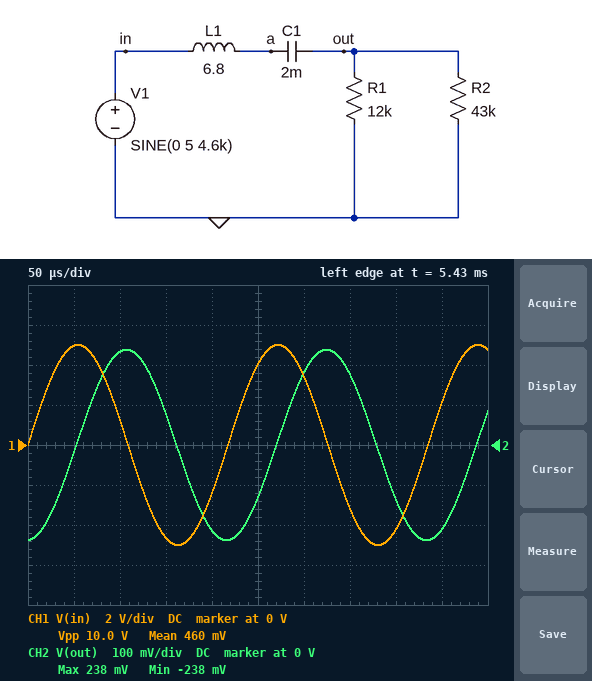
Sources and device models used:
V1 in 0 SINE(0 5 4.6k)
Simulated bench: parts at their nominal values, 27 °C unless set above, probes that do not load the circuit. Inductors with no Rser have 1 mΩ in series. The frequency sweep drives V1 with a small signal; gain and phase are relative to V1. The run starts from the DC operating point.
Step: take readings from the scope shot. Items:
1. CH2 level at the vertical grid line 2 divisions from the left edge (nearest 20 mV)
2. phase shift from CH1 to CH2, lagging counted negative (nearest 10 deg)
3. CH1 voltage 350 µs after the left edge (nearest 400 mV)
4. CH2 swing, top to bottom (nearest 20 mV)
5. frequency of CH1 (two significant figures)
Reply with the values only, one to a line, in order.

240 mV
-90 deg
-3.2 V
480 mV
4.6 kHz
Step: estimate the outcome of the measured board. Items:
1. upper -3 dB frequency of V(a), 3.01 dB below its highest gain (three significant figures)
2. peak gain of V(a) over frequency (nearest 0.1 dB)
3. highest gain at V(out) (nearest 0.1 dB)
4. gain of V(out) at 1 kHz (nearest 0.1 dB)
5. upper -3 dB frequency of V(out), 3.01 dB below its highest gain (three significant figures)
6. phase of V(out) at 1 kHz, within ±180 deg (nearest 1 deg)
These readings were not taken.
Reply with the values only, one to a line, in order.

220 Hz
0 dB
0 dB
-13.4 dB
220 Hz
-78 deg
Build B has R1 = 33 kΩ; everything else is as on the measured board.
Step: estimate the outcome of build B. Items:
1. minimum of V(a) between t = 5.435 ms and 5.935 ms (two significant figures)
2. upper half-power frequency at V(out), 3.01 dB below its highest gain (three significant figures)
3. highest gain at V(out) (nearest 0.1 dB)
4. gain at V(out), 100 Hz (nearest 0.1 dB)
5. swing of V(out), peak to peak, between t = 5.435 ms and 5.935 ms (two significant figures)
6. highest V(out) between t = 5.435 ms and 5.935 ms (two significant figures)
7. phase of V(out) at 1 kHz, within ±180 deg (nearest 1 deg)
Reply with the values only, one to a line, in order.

-470 mV
437 Hz
0 dB
-0.2 dB
950 mV
470 mV
-66 deg
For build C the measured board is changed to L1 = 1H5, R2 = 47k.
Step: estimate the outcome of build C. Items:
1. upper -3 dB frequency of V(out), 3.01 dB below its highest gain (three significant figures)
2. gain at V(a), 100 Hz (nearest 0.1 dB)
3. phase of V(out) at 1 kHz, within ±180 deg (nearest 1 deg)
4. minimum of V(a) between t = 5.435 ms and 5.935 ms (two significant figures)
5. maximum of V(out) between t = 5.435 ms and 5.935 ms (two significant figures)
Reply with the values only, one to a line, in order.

1.01 kHz
0 dB
-45 deg
-1.1 V
1.1 V
